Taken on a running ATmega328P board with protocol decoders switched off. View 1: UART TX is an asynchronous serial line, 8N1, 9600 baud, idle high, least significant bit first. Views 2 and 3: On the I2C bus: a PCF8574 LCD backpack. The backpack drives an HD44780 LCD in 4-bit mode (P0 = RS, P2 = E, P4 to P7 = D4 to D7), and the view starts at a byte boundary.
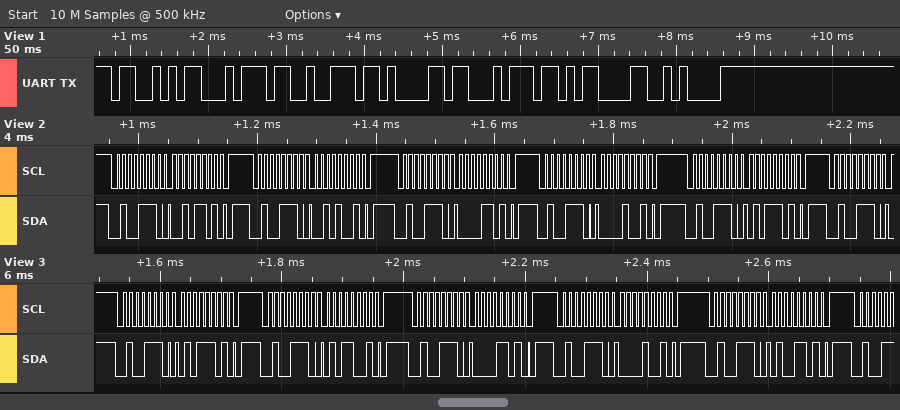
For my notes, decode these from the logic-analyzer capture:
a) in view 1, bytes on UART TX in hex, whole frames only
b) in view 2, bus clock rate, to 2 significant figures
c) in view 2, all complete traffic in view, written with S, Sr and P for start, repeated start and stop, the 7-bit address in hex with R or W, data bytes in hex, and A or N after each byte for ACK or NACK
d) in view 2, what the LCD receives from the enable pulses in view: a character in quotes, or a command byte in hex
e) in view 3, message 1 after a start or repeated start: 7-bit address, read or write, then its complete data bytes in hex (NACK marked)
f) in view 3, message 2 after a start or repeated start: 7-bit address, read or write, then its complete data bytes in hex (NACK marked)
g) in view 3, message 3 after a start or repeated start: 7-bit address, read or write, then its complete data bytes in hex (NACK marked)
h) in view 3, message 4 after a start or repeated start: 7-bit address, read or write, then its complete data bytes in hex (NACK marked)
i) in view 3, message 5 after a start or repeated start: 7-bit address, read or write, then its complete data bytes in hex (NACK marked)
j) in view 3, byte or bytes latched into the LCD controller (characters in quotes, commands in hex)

53 74 72 61 74 0D 0A
100 kHz
S 27W A 2D A P S 27W A 29 A P S 27W A 0D A P S 27W A 09 A P S 27W A 5D A P S 27W A
' '
0x27 write: 5D
0x27 write: 59
0x27 write: 0D
0x27 write: 09
0x27 write: 4D
'P'
